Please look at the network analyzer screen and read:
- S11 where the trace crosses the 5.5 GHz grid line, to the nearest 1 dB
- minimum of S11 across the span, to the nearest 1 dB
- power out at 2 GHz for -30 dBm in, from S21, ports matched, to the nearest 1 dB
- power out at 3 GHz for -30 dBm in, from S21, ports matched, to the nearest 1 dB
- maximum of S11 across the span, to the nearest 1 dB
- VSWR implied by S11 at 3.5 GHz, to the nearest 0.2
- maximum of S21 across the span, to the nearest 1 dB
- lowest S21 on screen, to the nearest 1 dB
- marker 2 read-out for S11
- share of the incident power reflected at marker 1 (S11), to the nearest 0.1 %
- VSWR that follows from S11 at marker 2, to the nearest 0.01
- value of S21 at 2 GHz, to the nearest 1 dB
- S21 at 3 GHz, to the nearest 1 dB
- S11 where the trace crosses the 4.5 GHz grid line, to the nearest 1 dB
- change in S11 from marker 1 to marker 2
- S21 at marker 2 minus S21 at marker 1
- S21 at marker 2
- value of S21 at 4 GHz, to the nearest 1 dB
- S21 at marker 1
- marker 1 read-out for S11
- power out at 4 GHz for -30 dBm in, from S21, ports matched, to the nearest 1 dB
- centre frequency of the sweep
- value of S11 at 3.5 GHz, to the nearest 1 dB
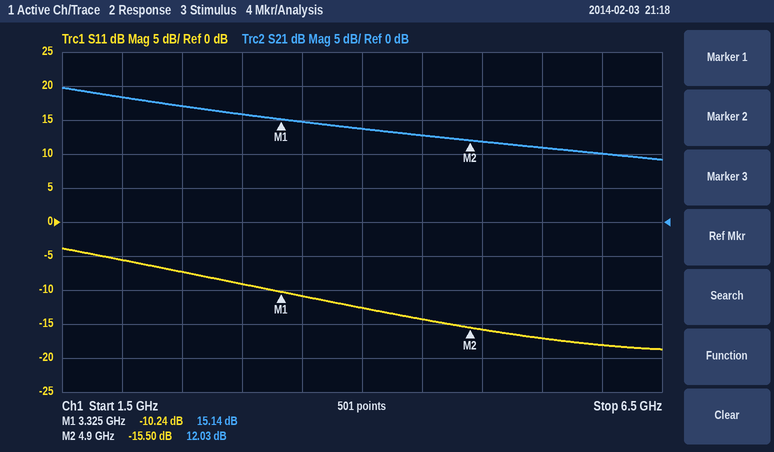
-17 dB
-19 dB
-12 dBm
-14 dBm
-4 dB
1.8
20 dB
9 dB
-15.50 dB
9.5 %
1.40
18 dB
16 dB
-14 dB
-5.26 dB
-3.11 dB
12.03 dB
14 dB
15.14 dB
-10.24 dB
-16 dBm
4 GHz
-11 dB
